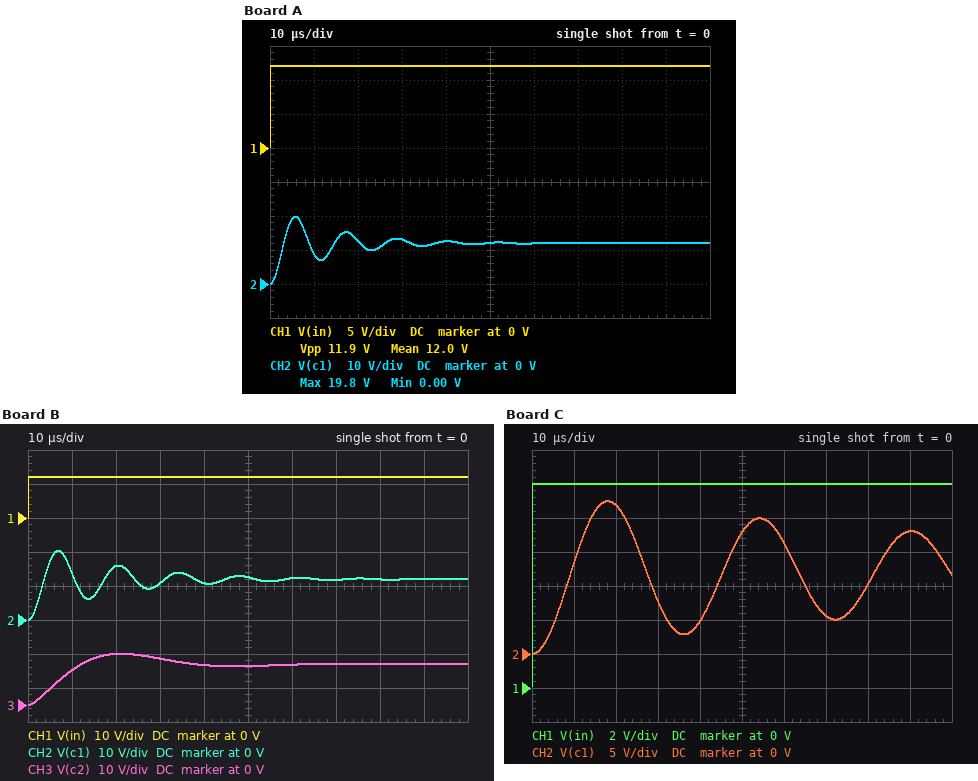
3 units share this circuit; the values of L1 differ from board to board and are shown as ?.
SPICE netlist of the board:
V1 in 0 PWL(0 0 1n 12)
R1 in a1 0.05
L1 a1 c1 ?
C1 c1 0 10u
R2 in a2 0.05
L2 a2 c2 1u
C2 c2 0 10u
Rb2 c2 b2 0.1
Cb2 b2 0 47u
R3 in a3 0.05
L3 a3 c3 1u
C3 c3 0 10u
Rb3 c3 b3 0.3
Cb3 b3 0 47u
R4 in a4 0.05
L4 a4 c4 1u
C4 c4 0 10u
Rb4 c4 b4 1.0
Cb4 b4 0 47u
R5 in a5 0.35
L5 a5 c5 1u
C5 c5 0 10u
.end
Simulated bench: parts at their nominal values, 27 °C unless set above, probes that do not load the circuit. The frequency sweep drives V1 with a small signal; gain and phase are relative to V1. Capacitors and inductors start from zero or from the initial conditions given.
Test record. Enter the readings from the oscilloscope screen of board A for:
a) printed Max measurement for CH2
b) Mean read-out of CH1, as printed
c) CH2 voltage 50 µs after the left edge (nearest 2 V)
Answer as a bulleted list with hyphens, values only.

- 19.8 V
- 12.0 V
- 12 V
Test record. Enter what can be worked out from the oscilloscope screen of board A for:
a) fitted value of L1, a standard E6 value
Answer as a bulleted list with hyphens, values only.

- 330 nH
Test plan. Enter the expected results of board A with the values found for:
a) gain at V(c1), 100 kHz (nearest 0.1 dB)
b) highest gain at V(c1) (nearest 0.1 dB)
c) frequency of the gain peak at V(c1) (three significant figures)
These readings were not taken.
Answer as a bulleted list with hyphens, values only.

- 7.2 dB
- 11.3 dB
- 85.9 kHz
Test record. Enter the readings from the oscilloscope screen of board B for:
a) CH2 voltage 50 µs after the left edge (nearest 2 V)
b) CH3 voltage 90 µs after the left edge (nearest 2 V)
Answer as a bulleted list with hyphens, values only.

- 12 V
- 12 V
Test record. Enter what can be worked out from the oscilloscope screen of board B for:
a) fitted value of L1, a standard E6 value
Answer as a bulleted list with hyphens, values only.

- 470 nH
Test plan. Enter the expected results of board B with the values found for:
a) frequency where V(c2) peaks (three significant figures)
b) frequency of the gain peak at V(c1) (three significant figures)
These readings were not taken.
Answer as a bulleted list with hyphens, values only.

- 18.0 kHz
- 72.4 kHz
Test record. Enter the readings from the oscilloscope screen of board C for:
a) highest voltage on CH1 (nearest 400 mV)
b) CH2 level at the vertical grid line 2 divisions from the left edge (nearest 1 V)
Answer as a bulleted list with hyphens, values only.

- 12.0 V
- 22 V
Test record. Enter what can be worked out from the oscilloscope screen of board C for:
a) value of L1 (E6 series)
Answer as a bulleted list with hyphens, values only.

- 3.3 µH
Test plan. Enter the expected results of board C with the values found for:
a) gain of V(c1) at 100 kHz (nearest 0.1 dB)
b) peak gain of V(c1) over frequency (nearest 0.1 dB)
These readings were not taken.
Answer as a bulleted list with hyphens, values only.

- -21.6 dB
- 21.2 dB
